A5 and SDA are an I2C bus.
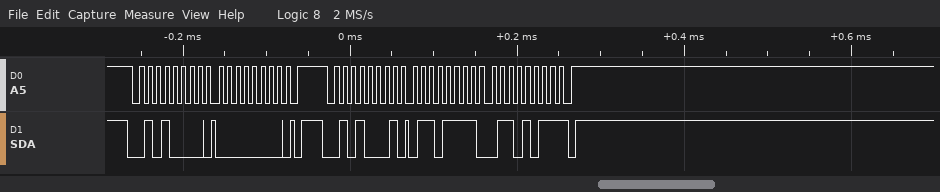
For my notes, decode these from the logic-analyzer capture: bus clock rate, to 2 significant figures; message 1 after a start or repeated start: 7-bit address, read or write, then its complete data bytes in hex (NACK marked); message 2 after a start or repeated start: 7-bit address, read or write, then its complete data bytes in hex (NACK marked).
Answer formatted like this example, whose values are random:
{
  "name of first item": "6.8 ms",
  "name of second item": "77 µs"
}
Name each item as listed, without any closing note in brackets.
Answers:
{
  "bus clock rate, to 2 significant figures": "100 kHz",
  "message 1 after a start or repeated start: 7-bit address, read or write, then its complete data bytes in hex": "0x28 write: 00",
  "message 2 after a start or repeated start: 7-bit address, read or write, then its complete data bytes in hex": "0x28 read: 6F 6B NACK"
}
